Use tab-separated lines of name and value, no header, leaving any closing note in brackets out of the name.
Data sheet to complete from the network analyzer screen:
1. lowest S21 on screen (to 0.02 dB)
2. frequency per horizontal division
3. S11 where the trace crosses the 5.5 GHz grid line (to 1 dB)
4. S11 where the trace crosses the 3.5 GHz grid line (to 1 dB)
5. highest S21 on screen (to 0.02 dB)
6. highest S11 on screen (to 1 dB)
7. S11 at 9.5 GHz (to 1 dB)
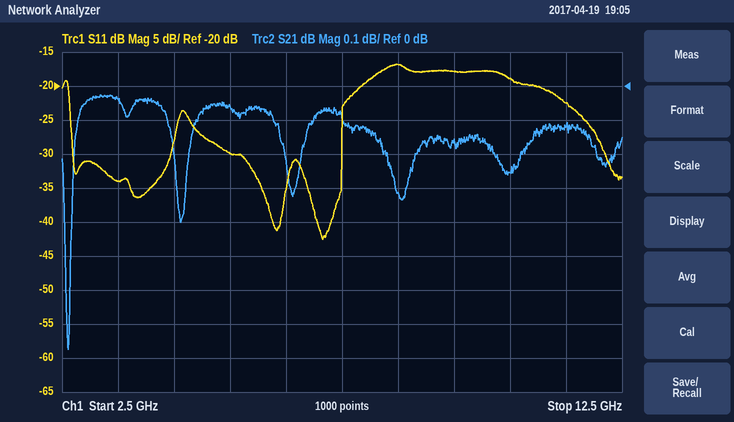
lowest S21 on screen	-0.78 dB
frequency per horizontal division	1 GHz
S11 where the trace crosses the 5.5 GHz grid line	-30 dB
S11 where the trace crosses the 3.5 GHz grid line	-34 dB
highest S21 on screen	-0.02 dB
highest S11 on screen	-17 dB
S11 at 9.5 GHz	-18 dB
